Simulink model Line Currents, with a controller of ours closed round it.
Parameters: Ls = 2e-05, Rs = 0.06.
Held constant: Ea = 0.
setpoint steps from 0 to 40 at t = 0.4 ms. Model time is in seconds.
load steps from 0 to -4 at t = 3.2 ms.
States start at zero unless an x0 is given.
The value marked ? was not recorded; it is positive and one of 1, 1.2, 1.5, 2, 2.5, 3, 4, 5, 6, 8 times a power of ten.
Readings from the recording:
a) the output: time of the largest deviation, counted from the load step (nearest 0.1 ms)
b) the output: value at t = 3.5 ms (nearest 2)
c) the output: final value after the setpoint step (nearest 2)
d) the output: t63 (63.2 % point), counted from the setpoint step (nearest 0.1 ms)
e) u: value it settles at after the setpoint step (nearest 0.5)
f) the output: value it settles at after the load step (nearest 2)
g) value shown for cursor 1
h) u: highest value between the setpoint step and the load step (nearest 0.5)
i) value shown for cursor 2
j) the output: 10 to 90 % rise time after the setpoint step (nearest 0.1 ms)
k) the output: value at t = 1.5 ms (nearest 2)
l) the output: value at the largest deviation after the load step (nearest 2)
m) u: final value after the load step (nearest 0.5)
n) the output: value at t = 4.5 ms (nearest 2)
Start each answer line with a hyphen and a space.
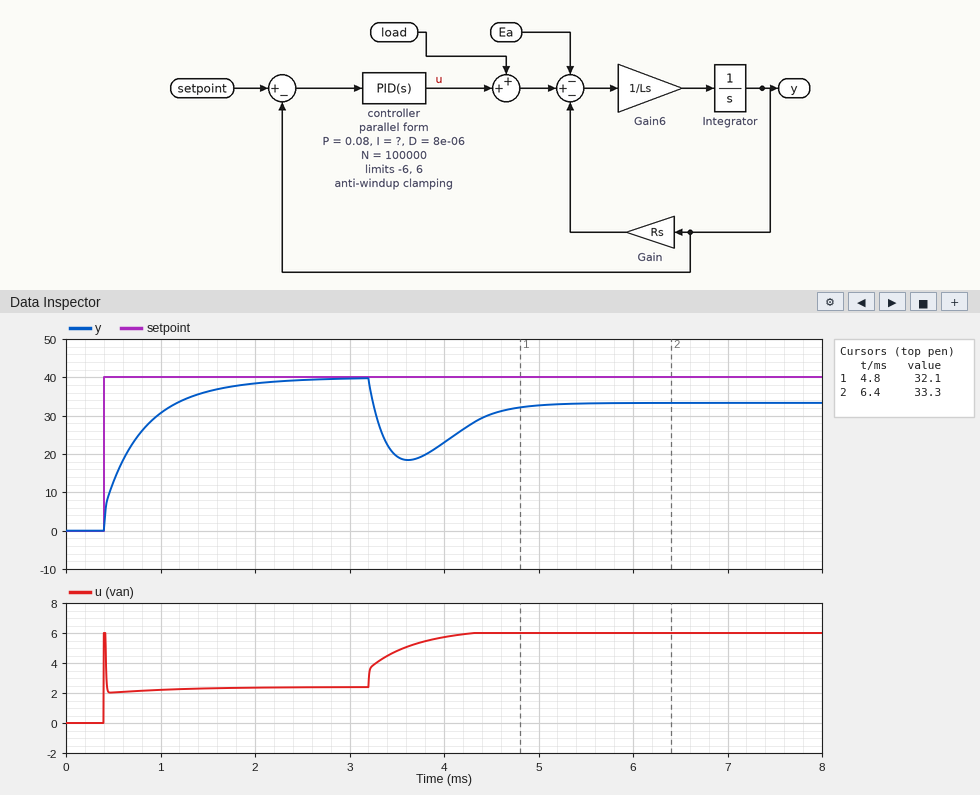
- 0.4 ms
- 20
- 40
- 0.4 ms
- 2.5
- 34
- 32.1
- 6.0
- 33.3
- 1.0 ms
- 36
- 18
- 6.0
- 30
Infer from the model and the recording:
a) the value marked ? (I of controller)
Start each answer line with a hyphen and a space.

- 150
